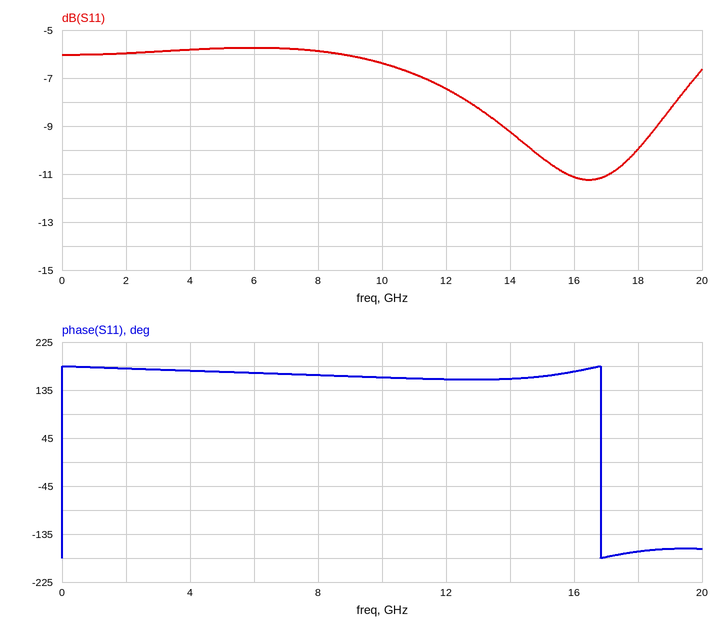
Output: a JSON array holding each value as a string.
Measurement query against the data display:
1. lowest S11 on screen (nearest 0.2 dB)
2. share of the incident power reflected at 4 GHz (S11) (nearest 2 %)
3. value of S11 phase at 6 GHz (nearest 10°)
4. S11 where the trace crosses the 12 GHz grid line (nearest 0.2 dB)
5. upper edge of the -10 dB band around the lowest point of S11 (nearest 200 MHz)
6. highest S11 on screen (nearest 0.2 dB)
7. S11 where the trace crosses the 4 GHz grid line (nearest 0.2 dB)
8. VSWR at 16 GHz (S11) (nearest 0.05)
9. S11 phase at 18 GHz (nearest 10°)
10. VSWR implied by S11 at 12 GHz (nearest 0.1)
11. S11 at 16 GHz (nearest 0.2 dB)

["-11.2 dB", "26 %", "170°", "-7.4 dB", "18.0 GHz", "-5.8 dB", "-5.8 dB", "1.75", "-170°", "2.5", "-11.2 dB"]
